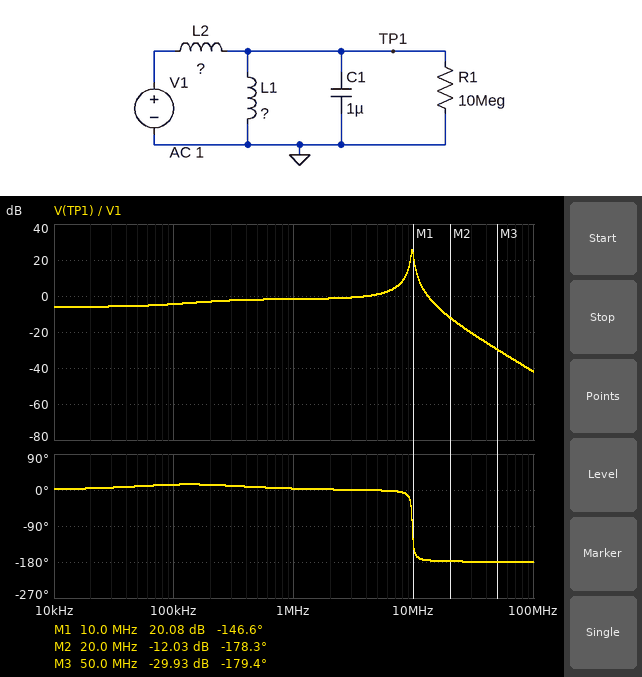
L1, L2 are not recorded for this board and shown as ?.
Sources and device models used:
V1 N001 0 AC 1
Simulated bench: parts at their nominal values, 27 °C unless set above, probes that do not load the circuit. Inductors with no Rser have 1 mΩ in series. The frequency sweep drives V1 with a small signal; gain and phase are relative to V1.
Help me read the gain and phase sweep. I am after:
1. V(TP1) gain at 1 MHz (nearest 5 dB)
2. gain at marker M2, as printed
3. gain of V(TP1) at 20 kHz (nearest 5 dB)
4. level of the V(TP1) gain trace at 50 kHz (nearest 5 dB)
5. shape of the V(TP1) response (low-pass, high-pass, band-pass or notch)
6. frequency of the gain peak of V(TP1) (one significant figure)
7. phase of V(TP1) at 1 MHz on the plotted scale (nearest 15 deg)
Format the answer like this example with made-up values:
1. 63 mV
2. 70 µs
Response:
1. 0 dB
2. -12.03 dB
3. -5 dB
4. -5 dB
5. band-pass
6. 10 MHz
7. 0 deg
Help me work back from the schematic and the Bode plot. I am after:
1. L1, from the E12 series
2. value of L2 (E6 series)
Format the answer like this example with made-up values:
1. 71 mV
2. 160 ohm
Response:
1. 1.5 nH
2. 330 pH
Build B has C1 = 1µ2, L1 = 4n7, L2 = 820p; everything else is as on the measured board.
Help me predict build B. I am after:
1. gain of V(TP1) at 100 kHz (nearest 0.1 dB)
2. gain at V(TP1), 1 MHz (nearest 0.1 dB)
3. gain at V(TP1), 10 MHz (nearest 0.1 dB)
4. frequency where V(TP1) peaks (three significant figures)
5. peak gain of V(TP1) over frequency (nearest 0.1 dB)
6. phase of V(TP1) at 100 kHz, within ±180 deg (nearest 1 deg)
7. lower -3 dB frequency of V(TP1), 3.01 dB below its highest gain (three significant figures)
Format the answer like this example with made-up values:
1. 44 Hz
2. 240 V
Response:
1. -2.2 dB
2. -1.1 dB
3. -8.7 dB
4. 5.50 MHz
5. 28.8 dB
6. 11 deg
7. 5.41 MHz
